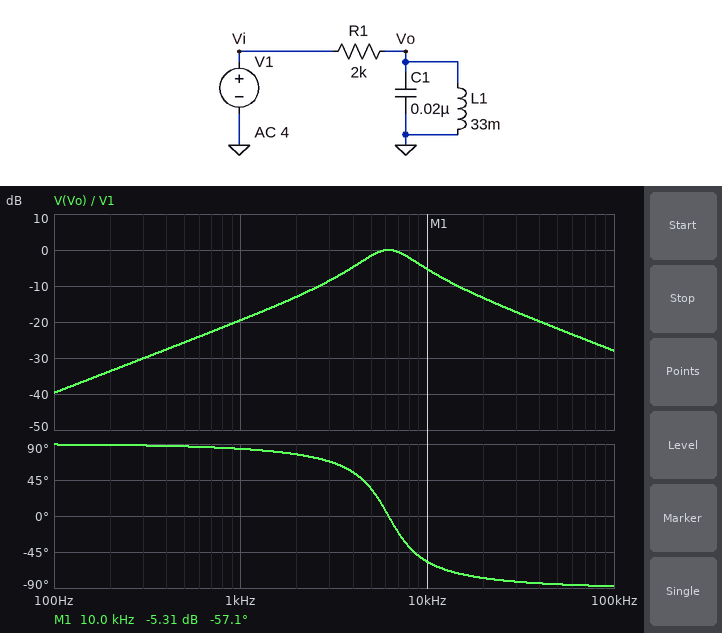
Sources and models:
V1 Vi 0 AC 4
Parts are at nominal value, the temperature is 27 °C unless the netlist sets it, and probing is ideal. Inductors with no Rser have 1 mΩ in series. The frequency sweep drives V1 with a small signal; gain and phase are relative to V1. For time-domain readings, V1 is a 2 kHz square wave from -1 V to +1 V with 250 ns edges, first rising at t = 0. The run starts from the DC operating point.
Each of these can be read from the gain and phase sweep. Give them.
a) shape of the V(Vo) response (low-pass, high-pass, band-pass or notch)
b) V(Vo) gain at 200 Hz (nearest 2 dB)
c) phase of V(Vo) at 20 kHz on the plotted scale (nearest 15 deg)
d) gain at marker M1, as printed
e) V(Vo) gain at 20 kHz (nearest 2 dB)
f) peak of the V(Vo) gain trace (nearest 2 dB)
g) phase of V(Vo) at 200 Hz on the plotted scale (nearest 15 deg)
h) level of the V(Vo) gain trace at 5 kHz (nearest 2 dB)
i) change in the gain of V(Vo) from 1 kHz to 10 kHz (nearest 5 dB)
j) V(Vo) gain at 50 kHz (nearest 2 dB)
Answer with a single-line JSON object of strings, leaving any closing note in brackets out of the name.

{"shape of the V(Vo) response": "band-pass", "V(Vo) gain at 200 Hz": "-34 dB", "phase of V(Vo) at 20 kHz on the plotted scale": "-75 deg", "gain at marker M1, as printed": "-5.31 dB", "V(Vo) gain at 20 kHz": "-14 dB", "peak of the V(Vo) gain trace": "0 dB", "phase of V(Vo) at 200 Hz on the plotted scale": "90 deg", "level of the V(Vo) gain trace at 5 kHz": "-2 dB", "change in the gain of V(Vo) from 1 kHz to 10 kHz": "15 dB", "V(Vo) gain at 50 kHz": "-22 dB"}
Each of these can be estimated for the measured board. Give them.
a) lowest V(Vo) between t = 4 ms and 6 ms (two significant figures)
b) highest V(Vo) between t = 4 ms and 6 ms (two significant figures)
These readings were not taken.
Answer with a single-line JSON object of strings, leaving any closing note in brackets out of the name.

{"lowest V(Vo) between t = 4 ms and 6 ms": "-880 mV", "highest V(Vo) between t = 4 ms and 6 ms": "880 mV"}
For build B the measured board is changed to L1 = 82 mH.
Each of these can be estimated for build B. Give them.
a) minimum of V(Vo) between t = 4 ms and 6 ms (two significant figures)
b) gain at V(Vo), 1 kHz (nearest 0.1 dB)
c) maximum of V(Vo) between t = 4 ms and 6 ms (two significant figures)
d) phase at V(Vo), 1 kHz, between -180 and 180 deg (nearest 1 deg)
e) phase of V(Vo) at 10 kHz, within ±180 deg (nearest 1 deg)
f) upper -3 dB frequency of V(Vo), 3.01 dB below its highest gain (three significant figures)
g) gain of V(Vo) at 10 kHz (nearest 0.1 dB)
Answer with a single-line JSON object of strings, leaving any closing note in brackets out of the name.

{"minimum of V(Vo) between t = 4 ms and 6 ms": "-1.1 V", "gain at V(Vo), 1 kHz": "-11.5 dB", "maximum of V(Vo) between t = 4 ms and 6 ms": "1.1 V", "phase at V(Vo), 1 kHz, between -180 and 180 deg": "75 deg", "phase of V(Vo) at 10 kHz, within ±180 deg": "-65 deg", "upper -3 dB frequency of V(Vo), 3.01 dB below its highest gain": "6.39 kHz", "gain of V(Vo) at 10 kHz": "-7.4 dB"}
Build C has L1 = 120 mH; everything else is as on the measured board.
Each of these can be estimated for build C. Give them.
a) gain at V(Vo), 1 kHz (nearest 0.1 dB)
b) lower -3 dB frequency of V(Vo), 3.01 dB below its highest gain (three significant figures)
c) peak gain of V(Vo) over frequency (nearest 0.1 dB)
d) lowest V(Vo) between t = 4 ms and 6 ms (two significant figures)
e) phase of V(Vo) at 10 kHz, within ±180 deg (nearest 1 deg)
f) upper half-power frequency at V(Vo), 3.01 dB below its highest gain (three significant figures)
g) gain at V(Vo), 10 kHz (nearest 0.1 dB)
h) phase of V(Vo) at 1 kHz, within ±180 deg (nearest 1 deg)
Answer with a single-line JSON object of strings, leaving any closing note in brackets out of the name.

{"gain at V(Vo), 1 kHz": "-8.3 dB", "lower -3 dB frequency of V(Vo), 3.01 dB below its highest gain": "1.82 kHz", "peak gain of V(Vo) over frequency": "0 dB", "lowest V(Vo) between t = 4 ms and 6 ms": "-1.3 V", "phase of V(Vo) at 10 kHz, within ±180 deg": "-66 deg", "upper half-power frequency at V(Vo), 3.01 dB below its highest gain": "5.80 kHz", "gain at V(Vo), 10 kHz": "-7.8 dB", "phase of V(Vo) at 1 kHz, within ±180 deg": "67 deg"}
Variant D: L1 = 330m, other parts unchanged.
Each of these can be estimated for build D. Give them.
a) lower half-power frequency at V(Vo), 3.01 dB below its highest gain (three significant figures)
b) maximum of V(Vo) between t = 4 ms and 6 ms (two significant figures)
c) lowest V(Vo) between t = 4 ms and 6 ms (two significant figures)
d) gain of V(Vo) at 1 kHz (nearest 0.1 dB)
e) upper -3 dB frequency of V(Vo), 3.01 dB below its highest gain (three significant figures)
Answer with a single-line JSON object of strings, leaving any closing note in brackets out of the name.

{"lower half-power frequency at V(Vo), 3.01 dB below its highest gain": "803 Hz", "maximum of V(Vo) between t = 4 ms and 6 ms": "1.2 V", "lowest V(Vo) between t = 4 ms and 6 ms": "-1.2 V", "gain of V(Vo) at 1 kHz": "-1.8 dB", "upper -3 dB frequency of V(Vo), 3.01 dB below its highest gain": "4.78 kHz"}
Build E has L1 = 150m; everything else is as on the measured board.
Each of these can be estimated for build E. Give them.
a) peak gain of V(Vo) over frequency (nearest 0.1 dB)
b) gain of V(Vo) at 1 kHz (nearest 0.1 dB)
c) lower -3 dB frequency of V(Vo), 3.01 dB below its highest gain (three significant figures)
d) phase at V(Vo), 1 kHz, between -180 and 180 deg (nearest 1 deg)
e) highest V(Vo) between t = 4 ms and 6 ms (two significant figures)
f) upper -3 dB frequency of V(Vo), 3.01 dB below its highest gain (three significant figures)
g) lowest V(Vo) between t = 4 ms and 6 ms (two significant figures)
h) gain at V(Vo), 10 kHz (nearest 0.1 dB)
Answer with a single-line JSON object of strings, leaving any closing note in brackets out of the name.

{"peak gain of V(Vo) over frequency": "0 dB", "gain of V(Vo) at 1 kHz": "-6.5 dB", "lower -3 dB frequency of V(Vo), 3.01 dB below its highest gain": "1.53 kHz", "phase at V(Vo), 1 kHz, between -180 and 180 deg": "62 deg", "highest V(Vo) between t = 4 ms and 6 ms": "1.3 V", "upper -3 dB frequency of V(Vo), 3.01 dB below its highest gain": "5.51 kHz", "lowest V(Vo) between t = 4 ms and 6 ms": "-1.3 V", "gain at V(Vo), 10 kHz": "-8.0 dB"}
